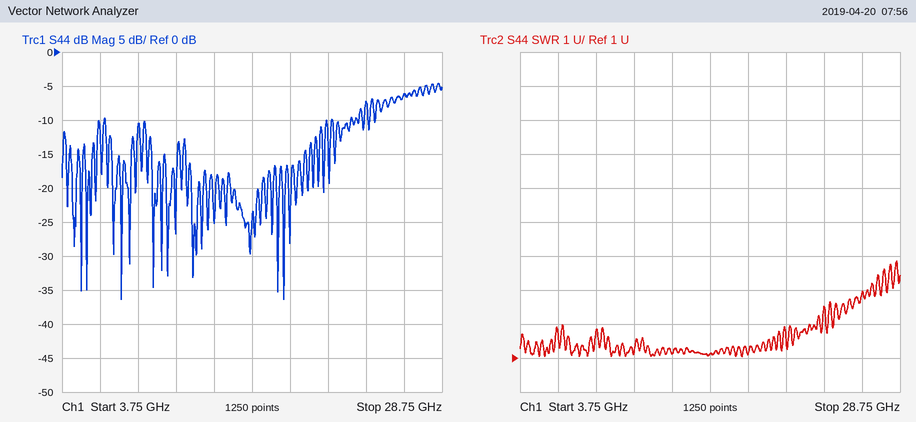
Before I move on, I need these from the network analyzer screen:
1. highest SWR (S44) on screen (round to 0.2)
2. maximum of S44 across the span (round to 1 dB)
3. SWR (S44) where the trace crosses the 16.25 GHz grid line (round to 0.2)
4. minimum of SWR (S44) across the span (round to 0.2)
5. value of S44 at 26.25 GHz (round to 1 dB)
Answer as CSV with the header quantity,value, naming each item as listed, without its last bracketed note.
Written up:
quantity,value
highest SWR (S44) on screen,3.8
maximum of S44 across the span,-5 dB
SWR (S44) where the trace crosses the 16.25 GHz grid line,1.2
minimum of SWR (S44) across the span,1.0
value of S44 at 26.25 GHz,-6 dB
